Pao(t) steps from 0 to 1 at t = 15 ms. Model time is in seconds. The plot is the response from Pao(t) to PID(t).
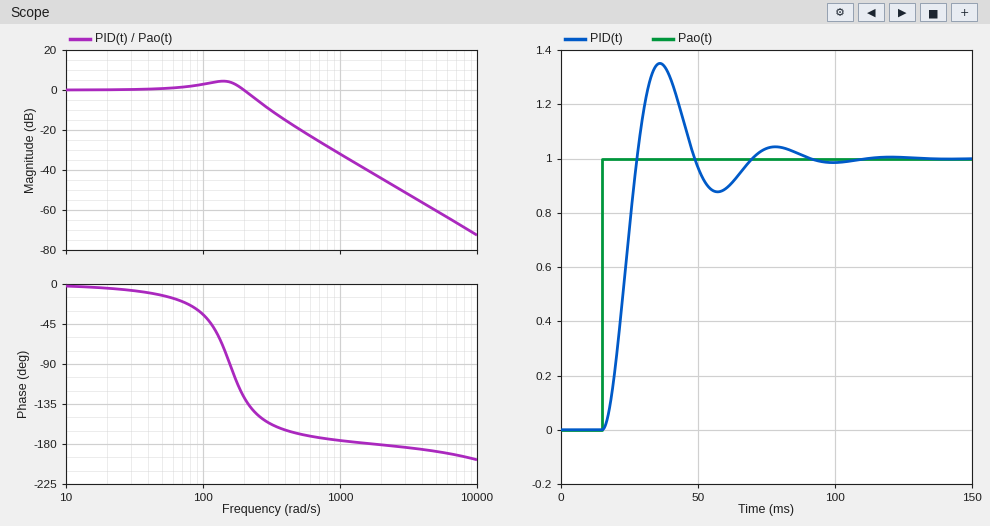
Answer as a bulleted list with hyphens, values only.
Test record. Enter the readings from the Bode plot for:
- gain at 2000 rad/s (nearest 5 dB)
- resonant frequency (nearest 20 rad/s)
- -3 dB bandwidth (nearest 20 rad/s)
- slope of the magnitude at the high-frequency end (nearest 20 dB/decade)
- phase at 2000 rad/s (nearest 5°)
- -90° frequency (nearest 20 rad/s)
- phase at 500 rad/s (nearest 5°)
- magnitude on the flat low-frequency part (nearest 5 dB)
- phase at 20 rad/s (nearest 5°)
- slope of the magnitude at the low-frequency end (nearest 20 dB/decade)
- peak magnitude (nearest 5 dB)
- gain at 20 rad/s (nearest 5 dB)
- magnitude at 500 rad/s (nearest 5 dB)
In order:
- -45 dB
- 140 rad/s
- 220 rad/s
- -40 dB/decade
- -180°
- 160 rad/s
- -170°
- 0 dB
- -5°
- 0 dB/decade
- 5 dB
- 0 dB
- -20 dB
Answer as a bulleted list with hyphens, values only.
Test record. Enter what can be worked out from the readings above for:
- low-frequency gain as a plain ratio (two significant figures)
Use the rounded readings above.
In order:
- 1.0
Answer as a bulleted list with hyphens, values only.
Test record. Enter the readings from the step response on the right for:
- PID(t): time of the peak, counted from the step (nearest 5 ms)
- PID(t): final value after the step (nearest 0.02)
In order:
- 20 ms
- 1.00
